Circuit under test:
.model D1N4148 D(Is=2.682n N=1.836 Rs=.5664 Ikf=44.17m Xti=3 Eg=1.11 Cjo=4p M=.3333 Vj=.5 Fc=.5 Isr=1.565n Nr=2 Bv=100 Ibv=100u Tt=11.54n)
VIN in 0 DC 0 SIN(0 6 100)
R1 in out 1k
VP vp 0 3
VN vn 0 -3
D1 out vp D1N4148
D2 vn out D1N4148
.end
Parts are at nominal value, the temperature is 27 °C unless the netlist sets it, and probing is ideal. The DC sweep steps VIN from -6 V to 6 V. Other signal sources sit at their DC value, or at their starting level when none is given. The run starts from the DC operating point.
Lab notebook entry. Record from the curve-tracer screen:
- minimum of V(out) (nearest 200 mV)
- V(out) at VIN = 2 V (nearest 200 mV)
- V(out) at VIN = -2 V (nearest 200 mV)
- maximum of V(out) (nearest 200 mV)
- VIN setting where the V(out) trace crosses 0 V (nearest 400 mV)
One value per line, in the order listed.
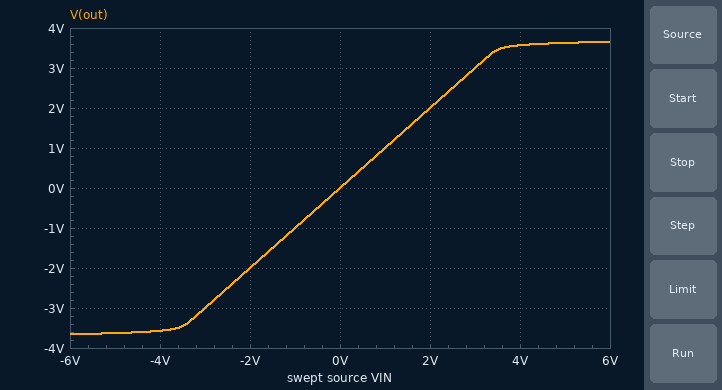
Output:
-3.6 V
2.0 V
-2.0 V
3.6 V
0 V
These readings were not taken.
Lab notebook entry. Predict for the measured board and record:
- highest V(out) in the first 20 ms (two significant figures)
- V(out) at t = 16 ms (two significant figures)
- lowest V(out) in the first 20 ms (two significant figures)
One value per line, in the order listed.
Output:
3.7 V
-3.5 V
-3.7 V
